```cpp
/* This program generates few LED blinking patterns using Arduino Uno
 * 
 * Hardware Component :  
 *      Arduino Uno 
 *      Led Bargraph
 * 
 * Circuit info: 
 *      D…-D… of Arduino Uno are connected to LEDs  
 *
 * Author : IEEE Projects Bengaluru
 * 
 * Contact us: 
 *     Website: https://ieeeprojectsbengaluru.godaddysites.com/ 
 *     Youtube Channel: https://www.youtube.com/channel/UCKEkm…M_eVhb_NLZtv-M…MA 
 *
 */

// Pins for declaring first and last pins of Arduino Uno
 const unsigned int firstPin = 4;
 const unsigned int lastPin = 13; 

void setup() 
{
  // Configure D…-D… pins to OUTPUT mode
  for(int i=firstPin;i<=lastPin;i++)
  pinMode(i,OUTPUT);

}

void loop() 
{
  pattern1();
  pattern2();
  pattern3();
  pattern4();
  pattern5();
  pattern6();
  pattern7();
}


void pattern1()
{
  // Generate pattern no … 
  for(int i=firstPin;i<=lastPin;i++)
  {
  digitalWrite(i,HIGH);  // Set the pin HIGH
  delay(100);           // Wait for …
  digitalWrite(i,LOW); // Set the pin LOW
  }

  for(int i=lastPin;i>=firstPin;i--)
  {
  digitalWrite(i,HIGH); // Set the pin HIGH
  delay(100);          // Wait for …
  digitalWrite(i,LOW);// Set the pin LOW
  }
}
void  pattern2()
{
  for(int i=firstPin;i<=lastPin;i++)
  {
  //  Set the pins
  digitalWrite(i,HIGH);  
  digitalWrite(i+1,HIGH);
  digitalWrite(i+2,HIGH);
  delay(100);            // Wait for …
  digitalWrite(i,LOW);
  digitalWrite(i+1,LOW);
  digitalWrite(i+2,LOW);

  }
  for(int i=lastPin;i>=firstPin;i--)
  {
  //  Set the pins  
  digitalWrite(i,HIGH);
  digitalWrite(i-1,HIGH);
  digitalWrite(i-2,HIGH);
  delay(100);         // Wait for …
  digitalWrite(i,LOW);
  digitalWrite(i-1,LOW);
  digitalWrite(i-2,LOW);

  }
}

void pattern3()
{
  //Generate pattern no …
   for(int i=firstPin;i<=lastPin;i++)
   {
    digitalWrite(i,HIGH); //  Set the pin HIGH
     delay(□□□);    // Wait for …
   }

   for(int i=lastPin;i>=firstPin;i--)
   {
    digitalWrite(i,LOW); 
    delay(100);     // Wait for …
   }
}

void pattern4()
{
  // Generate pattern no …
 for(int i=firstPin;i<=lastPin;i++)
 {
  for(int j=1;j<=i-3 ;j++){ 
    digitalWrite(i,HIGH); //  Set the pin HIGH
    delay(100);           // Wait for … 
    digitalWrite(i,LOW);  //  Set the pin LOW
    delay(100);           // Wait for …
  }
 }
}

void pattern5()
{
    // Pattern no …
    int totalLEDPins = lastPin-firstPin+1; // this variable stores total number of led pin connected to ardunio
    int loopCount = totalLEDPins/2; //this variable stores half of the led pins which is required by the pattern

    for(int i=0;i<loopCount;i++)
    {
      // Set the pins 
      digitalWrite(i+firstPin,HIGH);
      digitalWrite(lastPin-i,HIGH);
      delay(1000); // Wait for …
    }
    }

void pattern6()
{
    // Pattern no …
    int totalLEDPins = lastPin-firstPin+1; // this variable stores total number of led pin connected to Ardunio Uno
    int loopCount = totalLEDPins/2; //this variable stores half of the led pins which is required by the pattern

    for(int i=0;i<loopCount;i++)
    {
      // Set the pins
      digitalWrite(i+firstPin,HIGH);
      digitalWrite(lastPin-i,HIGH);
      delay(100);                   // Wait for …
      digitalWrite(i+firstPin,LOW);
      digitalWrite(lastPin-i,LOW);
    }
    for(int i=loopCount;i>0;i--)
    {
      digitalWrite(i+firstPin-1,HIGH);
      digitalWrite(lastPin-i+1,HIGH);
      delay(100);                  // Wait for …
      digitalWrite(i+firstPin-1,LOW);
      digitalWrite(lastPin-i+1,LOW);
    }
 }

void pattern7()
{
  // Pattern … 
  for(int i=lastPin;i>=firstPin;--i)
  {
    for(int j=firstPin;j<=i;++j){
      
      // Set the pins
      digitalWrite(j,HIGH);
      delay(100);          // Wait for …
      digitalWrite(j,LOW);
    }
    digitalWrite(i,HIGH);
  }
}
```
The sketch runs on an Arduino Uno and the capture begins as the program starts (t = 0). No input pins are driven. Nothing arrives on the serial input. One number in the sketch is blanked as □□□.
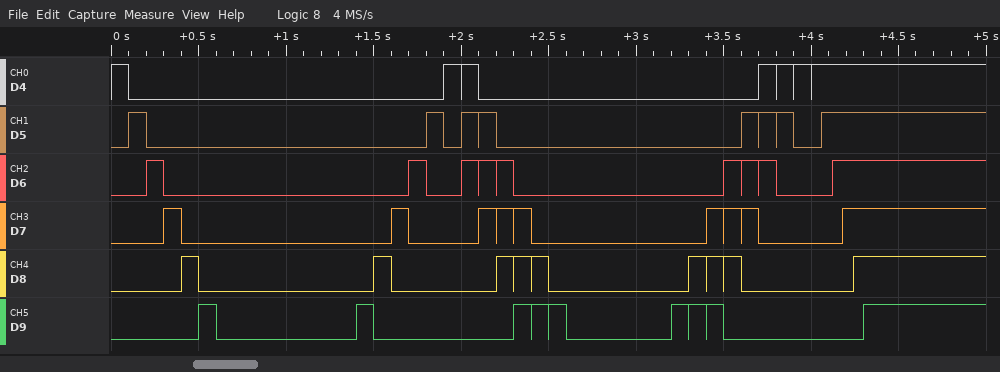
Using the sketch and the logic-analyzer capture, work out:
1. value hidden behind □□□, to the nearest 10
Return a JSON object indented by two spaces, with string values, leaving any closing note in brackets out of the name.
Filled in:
{
  "value hidden behind □□□, to the nearest 10": "60"
}
